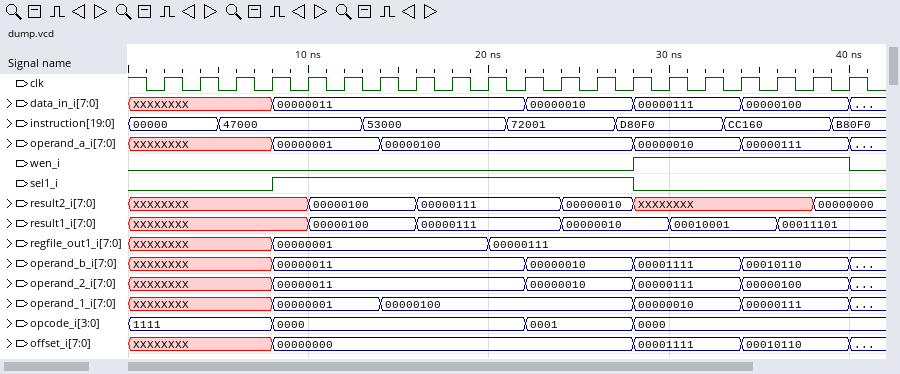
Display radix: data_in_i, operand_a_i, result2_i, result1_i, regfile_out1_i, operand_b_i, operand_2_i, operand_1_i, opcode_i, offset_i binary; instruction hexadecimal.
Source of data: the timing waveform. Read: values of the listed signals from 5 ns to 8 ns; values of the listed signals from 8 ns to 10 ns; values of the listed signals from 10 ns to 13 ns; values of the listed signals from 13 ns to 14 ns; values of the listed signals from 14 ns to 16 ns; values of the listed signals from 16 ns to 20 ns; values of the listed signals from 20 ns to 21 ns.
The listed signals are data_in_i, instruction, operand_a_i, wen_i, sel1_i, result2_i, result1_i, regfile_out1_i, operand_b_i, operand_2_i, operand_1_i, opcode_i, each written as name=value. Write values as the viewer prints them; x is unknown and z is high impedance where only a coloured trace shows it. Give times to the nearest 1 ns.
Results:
data_in_i=XXXXXXXX, instruction=47000, operand_a_i=XXXXXXXX, wen_i=0, sel1_i=0, result2_i=XXXXXXXX, result1_i=XXXXXXXX, regfile_out1_i=XXXXXXXX, operand_b_i=XXXXXXXX, operand_2_i=XXXXXXXX, operand_1_i=XXXXXXXX, opcode_i=1111
data_in_i=00000011, instruction=47000, operand_a_i=00000001, wen_i=0, sel1_i=1, result2_i=XXXXXXXX, result1_i=XXXXXXXX, regfile_out1_i=00000001, operand_b_i=00000011, operand_2_i=00000011, operand_1_i=00000001, opcode_i=0000
data_in_i=00000011, instruction=47000, operand_a_i=00000001, wen_i=0, sel1_i=1, result2_i=00000100, result1_i=00000100, regfile_out1_i=00000001, operand_b_i=00000011, operand_2_i=00000011, operand_1_i=00000001, opcode_i=0000
data_in_i=00000011, instruction=53000, operand_a_i=00000001, wen_i=0, sel1_i=1, result2_i=00000100, result1_i=00000100, regfile_out1_i=00000001, operand_b_i=00000011, operand_2_i=00000011, operand_1_i=00000001, opcode_i=0000
data_in_i=00000011, instruction=53000, operand_a_i=00000100, wen_i=0, sel1_i=1, result2_i=00000100, result1_i=00000100, regfile_out1_i=00000001, operand_b_i=00000011, operand_2_i=00000011, operand_1_i=00000100, opcode_i=0000
data_in_i=00000011, instruction=53000, operand_a_i=00000100, wen_i=0, sel1_i=1, result2_i=00000111, result1_i=00000111, regfile_out1_i=00000001, operand_b_i=00000011, operand_2_i=00000011, operand_1_i=00000100, opcode_i=0000
data_in_i=00000011, instruction=53000, operand_a_i=00000100, wen_i=0, sel1_i=1, result2_i=00000111, result1_i=00000111, regfile_out1_i=00000111, operand_b_i=00000011, operand_2_i=00000011, operand_1_i=00000100, opcode_i=0000
